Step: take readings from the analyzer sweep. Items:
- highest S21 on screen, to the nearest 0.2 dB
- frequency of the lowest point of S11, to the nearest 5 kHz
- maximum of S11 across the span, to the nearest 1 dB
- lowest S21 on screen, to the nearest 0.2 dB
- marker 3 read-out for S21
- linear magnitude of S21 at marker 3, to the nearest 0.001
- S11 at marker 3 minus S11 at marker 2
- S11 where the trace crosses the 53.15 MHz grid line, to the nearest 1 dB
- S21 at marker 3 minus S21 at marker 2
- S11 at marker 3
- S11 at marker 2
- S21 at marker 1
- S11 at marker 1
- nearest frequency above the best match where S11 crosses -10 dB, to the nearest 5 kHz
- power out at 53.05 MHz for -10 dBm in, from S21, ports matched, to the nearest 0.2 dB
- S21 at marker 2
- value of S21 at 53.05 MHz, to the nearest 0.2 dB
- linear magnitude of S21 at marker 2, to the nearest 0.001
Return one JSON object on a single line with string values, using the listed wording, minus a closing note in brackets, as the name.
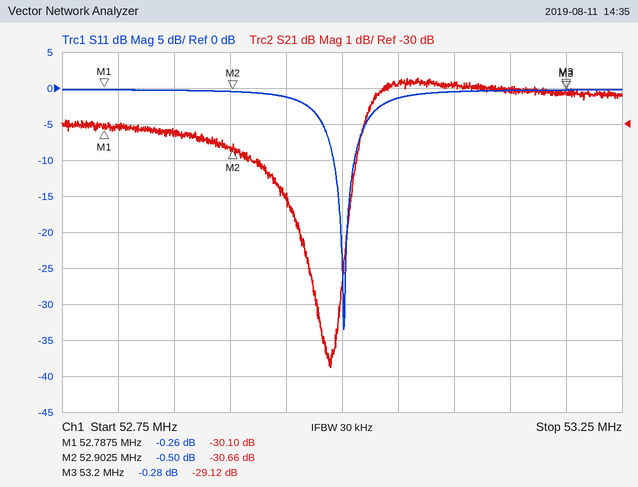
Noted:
{"highest S21 on screen, to the nearest 0.2 dB": "-28.8 dB", "frequency of the lowest point of S11, to the nearest 5 kHz": "53.000 MHz", "maximum of S11 across the span, to the nearest 1 dB": "0 dB", "lowest S21 on screen, to the nearest 0.2 dB": "-36.8 dB", "marker 3 read-out for S21": "-29.12 dB", "linear magnitude of S21 at marker 3, to the nearest 0.001": "0.035", "S11 at marker 3 minus S11 at marker 2": "0.22 dB", "S11 where the trace crosses the 53.15 MHz grid line, to the nearest 1 dB": "0 dB", "S21 at marker 3 minus S21 at marker 2": "1.54 dB", "S11 at marker 3": "-0.28 dB", "S11 at marker 2": "-0.50 dB", "S21 at marker 1": "-30.10 dB", "S11 at marker 1": "-0.26 dB", "nearest frequency above the best match where S11 crosses -10 dB, to the nearest 5 kHz": "53.010 MHz", "power out at 53.05 MHz for -10 dBm in, from S21, ports matched, to the nearest 0.2 dB": "-38.8 dBm", "S21 at marker 2": "-30.66 dB", "value of S21 at 53.05 MHz, to the nearest 0.2 dB": "-28.8 dB", "linear magnitude of S21 at marker 2, to the nearest 0.001": "0.029"}
